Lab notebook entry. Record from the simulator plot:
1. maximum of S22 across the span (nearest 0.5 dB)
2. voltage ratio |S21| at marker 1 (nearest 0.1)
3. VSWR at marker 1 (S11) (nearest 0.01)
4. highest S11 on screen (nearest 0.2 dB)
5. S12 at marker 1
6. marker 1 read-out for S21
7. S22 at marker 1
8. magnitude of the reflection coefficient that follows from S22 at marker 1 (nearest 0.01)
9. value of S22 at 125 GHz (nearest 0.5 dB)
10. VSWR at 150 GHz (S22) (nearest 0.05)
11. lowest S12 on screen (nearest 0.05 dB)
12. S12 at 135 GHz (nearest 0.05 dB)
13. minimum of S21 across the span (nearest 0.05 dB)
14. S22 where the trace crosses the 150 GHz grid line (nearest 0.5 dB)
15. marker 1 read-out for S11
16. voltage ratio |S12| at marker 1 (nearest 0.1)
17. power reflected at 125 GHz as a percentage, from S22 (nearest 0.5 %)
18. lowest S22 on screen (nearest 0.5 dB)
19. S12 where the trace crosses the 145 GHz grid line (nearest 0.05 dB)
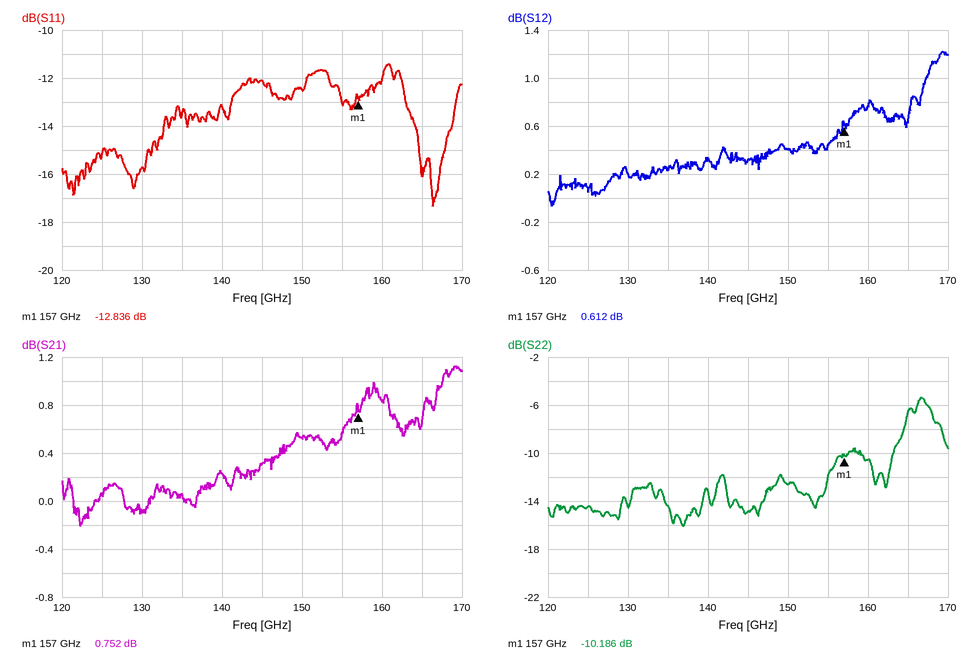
-5.5 dB
1.1
1.59
-11.4 dB
0.612 dB
0.752 dB
-10.186 dB
0.31
-14.5 dB
1.60
-0.05 dB
0.25 dB
-0.20 dB
-12.5 dB
-12.836 dB
1.1
3.5 %
-16.0 dB
0.30 dB
